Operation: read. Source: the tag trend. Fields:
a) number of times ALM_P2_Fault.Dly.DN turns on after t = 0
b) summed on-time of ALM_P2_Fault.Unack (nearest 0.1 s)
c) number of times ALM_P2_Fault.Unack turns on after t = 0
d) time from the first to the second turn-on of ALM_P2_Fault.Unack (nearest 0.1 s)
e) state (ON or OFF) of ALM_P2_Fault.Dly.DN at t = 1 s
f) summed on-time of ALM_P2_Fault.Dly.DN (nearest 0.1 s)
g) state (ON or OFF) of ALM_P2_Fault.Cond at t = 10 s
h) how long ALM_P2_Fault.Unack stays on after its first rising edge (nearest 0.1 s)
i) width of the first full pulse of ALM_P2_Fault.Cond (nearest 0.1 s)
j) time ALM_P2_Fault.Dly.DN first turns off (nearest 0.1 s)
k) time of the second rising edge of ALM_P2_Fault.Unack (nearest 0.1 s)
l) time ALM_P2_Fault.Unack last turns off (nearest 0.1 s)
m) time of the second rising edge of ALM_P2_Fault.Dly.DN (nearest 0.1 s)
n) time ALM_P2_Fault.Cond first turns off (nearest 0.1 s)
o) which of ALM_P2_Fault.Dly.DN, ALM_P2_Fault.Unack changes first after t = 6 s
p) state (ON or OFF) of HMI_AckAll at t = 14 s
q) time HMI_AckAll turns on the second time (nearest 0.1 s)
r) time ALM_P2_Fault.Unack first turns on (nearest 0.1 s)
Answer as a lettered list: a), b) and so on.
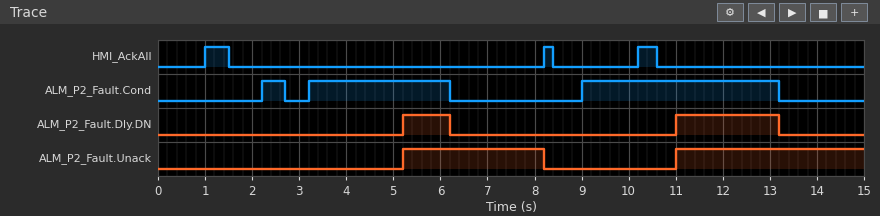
a) 2
b) 7.0 s
c) 2
d) 5.8 s
e) OFF
f) 3.2 s
g) ON
h) 3.0 s
i) 0.5 s
j) 6.2 s
k) 11.0 s
l) 8.2 s
m) 11.0 s
n) 2.7 s
o) ALM_P2_Fault.Dly.DN
p) OFF
q) 8.2 s
r) 5.2 s
